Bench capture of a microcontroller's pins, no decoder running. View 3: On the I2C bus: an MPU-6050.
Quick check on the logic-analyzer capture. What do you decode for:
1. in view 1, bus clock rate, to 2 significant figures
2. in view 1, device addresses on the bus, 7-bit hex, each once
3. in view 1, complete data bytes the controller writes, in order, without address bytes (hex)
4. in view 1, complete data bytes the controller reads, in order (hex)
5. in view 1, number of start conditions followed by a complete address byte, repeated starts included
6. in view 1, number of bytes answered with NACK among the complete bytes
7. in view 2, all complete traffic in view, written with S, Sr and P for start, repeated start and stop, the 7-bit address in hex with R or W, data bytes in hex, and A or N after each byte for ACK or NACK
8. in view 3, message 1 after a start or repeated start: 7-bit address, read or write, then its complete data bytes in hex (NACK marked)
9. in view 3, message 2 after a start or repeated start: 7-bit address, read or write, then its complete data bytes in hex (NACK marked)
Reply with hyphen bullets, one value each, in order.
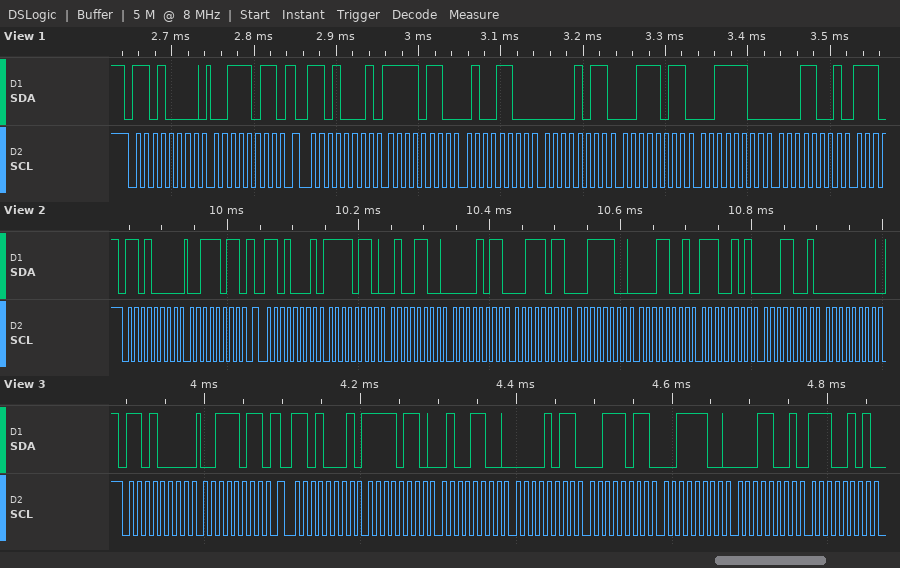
- 100 kHz
- 0x68
- 3B
- F6 4C 0B 3B 3C 19
- 2
- 0
- S 68W A 3B A Sr 68R A F6 A 4C A 0B A 3B A 3C A 19 A E5 A 19 A 00 A
- 0x68 write: 3B
- 0x68 read: F6 4C 0B 3B 3C 19 E5
